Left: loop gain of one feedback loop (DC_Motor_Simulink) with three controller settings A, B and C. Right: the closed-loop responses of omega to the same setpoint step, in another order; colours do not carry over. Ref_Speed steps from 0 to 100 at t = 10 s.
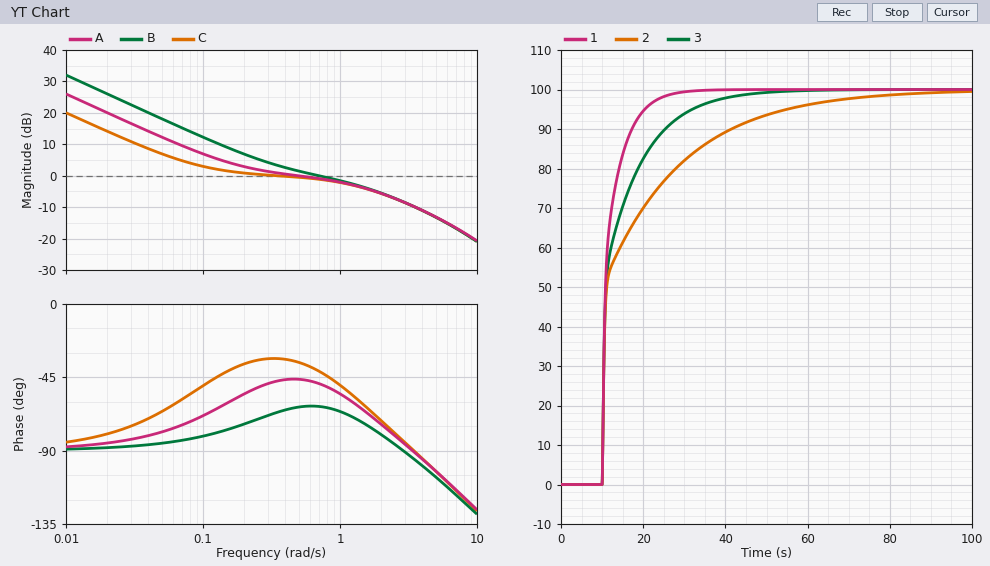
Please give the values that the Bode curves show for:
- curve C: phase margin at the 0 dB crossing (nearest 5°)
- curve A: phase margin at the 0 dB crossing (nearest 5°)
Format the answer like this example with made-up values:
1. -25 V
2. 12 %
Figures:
1. 145°
2. 135°
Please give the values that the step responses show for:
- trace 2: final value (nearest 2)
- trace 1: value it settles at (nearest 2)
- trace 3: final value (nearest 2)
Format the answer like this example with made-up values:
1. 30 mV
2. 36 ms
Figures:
1. 100
2. 100
3. 100
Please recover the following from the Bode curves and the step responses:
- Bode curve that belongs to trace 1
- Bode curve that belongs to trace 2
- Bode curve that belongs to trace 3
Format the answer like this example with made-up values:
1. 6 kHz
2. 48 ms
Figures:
1. B
2. C
3. A
